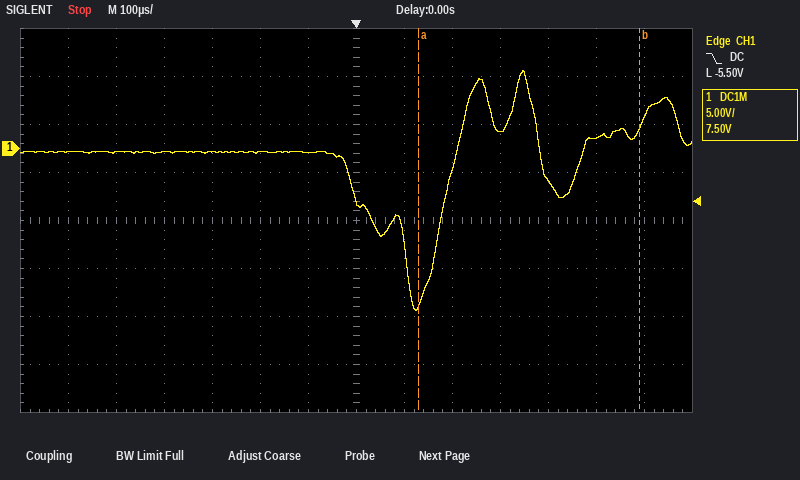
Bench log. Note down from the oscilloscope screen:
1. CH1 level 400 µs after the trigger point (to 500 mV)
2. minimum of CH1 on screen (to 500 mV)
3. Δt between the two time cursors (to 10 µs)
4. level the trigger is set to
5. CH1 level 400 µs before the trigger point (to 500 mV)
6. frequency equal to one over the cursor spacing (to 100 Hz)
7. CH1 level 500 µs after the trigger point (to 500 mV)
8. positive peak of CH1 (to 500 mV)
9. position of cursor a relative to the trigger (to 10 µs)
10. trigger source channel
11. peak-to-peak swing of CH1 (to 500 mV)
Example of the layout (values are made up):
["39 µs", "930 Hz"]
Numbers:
["-3.5 V", "-17.0 V", "460 µs", "-5.50 V", "-500 mV", "2.2 kHz", "1.0 V", "8.0 V", "+130 µs", "CH1", "25.0 V"]
